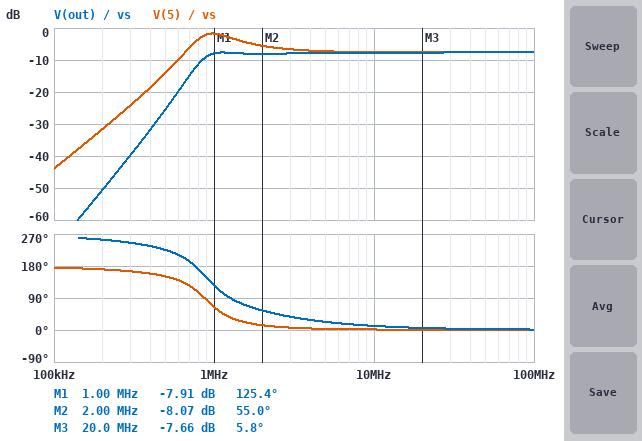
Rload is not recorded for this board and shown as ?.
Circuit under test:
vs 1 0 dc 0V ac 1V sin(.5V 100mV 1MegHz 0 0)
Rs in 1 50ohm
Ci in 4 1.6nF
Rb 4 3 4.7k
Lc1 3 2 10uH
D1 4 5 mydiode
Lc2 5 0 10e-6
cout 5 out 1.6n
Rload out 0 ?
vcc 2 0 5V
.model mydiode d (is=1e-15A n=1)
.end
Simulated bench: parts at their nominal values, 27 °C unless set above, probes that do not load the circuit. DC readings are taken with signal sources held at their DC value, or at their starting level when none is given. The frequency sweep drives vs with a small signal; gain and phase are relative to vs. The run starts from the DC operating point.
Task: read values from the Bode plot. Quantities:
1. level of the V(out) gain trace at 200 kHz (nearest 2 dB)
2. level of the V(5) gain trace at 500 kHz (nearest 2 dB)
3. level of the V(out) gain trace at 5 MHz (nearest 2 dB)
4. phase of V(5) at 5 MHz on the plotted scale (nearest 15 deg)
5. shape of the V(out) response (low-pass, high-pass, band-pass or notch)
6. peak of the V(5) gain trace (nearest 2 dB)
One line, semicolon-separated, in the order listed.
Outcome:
-50 dB; -14 dB; -8 dB; 0 deg; high-pass; -2 dB
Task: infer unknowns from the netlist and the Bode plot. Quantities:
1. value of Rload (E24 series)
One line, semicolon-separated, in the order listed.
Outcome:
56 Ω
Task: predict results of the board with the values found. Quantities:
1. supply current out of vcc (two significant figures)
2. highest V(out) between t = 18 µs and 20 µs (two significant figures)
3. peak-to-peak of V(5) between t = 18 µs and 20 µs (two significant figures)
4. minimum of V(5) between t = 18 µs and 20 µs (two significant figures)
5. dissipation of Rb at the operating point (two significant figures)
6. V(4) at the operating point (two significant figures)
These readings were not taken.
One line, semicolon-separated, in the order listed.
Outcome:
910 µA; 36 mV; 160 mV; -80 mV; 3.9 mW; 710 mV
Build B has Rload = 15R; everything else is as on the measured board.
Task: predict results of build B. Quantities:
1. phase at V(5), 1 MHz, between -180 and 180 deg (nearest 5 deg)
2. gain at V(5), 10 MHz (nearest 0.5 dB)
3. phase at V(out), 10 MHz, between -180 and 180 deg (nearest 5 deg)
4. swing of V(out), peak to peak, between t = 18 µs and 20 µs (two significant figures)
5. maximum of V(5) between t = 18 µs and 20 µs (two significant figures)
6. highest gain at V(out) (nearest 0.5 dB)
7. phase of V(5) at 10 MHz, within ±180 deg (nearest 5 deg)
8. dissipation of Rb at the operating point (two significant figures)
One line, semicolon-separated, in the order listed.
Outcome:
50 deg; -14.5 dB; 15 deg; 35 mV; 110 mV; -15.0 dB; -20 deg; 3.9 mW
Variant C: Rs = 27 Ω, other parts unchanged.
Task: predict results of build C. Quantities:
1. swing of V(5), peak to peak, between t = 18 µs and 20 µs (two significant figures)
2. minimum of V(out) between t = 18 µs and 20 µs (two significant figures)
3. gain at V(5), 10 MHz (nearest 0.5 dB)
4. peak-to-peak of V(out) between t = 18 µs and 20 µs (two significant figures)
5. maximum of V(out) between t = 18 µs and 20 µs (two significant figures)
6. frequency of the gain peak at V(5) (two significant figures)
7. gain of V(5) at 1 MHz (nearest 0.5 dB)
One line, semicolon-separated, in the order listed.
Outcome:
190 mV; -48 mV; -6.0 dB; 88 mV; 40 mV; 950 kHz; 0 dB
